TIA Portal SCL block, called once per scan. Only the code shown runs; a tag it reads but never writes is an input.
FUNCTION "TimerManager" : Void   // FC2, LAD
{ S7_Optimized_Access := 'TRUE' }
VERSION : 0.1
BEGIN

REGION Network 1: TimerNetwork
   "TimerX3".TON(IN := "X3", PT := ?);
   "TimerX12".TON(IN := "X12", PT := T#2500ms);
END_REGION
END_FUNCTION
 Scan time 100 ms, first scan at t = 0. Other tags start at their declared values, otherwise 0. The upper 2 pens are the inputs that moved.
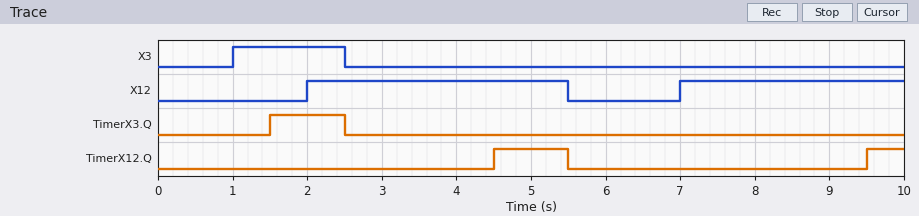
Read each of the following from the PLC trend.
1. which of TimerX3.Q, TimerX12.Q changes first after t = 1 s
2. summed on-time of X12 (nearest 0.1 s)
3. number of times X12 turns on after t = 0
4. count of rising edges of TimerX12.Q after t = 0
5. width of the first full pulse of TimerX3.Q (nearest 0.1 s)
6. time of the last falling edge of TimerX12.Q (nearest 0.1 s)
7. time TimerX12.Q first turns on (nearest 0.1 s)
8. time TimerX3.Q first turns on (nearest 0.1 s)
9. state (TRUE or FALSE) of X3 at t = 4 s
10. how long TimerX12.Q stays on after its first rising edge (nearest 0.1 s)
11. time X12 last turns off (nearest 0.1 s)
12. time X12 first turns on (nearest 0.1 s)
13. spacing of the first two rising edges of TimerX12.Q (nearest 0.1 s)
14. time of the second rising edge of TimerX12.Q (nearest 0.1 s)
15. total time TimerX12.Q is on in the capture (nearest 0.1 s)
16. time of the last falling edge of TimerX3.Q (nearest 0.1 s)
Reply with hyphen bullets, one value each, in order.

- TimerX3.Q
- 6.5 s
- 2
- 2
- 1.0 s
- 5.5 s
- 4.5 s
- 1.5 s
- FALSE
- 1.0 s
- 5.5 s
- 2.0 s
- 5.0 s
- 9.5 s
- 1.5 s
- 2.5 s
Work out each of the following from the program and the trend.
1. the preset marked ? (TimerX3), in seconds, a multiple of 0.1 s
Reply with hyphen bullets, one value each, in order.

- 0.5 s
